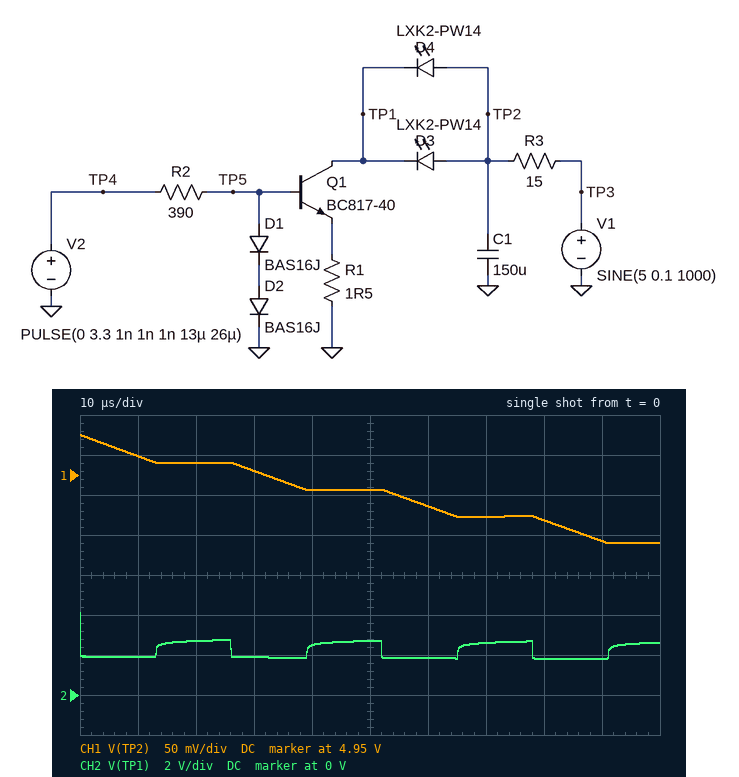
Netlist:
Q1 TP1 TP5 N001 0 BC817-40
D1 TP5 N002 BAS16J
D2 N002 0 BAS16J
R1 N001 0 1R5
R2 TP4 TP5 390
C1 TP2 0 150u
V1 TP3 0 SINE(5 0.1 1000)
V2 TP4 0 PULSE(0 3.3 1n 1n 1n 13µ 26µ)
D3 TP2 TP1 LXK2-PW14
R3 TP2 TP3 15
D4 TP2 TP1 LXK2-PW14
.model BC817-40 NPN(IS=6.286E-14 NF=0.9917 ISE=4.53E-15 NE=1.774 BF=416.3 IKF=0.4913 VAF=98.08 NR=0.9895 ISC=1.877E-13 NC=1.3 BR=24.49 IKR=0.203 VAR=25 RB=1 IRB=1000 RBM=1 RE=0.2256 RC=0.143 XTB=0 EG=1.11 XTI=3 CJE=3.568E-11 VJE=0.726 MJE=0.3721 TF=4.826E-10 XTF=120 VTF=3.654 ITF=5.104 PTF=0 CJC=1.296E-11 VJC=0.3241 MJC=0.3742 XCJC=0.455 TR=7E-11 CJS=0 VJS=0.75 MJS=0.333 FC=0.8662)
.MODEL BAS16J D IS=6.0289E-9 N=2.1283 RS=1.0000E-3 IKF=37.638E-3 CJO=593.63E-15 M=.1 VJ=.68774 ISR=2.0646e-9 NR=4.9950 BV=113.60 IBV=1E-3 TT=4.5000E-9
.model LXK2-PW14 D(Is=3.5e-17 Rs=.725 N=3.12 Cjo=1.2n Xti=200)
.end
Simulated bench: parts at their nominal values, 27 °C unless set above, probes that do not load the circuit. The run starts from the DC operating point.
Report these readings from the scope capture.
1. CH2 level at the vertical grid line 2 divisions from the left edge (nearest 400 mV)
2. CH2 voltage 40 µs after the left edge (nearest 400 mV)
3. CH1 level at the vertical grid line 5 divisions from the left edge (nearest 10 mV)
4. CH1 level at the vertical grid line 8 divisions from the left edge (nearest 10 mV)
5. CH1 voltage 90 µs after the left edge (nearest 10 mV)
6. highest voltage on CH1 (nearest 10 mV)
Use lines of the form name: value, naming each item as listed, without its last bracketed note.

CH2 level at the vertical grid line 2 divisions from the left edge: 2.8 V
CH2 voltage 40 µs after the left edge: 2.4 V
CH1 level at the vertical grid line 5 divisions from the left edge: 4.93 V
CH1 level at the vertical grid line 8 divisions from the left edge: 4.89 V
CH1 voltage 90 µs after the left edge: 4.87 V
highest voltage on CH1: 5.00 V
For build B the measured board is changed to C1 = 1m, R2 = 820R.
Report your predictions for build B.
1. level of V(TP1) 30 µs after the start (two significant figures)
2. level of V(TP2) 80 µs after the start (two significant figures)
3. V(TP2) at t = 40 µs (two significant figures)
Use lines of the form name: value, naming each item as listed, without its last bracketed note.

level of V(TP1) 30 µs after the start: 2.0 V
level of V(TP2) 80 µs after the start: 5.0 V
V(TP2) at t = 40 µs: 5.0 V
